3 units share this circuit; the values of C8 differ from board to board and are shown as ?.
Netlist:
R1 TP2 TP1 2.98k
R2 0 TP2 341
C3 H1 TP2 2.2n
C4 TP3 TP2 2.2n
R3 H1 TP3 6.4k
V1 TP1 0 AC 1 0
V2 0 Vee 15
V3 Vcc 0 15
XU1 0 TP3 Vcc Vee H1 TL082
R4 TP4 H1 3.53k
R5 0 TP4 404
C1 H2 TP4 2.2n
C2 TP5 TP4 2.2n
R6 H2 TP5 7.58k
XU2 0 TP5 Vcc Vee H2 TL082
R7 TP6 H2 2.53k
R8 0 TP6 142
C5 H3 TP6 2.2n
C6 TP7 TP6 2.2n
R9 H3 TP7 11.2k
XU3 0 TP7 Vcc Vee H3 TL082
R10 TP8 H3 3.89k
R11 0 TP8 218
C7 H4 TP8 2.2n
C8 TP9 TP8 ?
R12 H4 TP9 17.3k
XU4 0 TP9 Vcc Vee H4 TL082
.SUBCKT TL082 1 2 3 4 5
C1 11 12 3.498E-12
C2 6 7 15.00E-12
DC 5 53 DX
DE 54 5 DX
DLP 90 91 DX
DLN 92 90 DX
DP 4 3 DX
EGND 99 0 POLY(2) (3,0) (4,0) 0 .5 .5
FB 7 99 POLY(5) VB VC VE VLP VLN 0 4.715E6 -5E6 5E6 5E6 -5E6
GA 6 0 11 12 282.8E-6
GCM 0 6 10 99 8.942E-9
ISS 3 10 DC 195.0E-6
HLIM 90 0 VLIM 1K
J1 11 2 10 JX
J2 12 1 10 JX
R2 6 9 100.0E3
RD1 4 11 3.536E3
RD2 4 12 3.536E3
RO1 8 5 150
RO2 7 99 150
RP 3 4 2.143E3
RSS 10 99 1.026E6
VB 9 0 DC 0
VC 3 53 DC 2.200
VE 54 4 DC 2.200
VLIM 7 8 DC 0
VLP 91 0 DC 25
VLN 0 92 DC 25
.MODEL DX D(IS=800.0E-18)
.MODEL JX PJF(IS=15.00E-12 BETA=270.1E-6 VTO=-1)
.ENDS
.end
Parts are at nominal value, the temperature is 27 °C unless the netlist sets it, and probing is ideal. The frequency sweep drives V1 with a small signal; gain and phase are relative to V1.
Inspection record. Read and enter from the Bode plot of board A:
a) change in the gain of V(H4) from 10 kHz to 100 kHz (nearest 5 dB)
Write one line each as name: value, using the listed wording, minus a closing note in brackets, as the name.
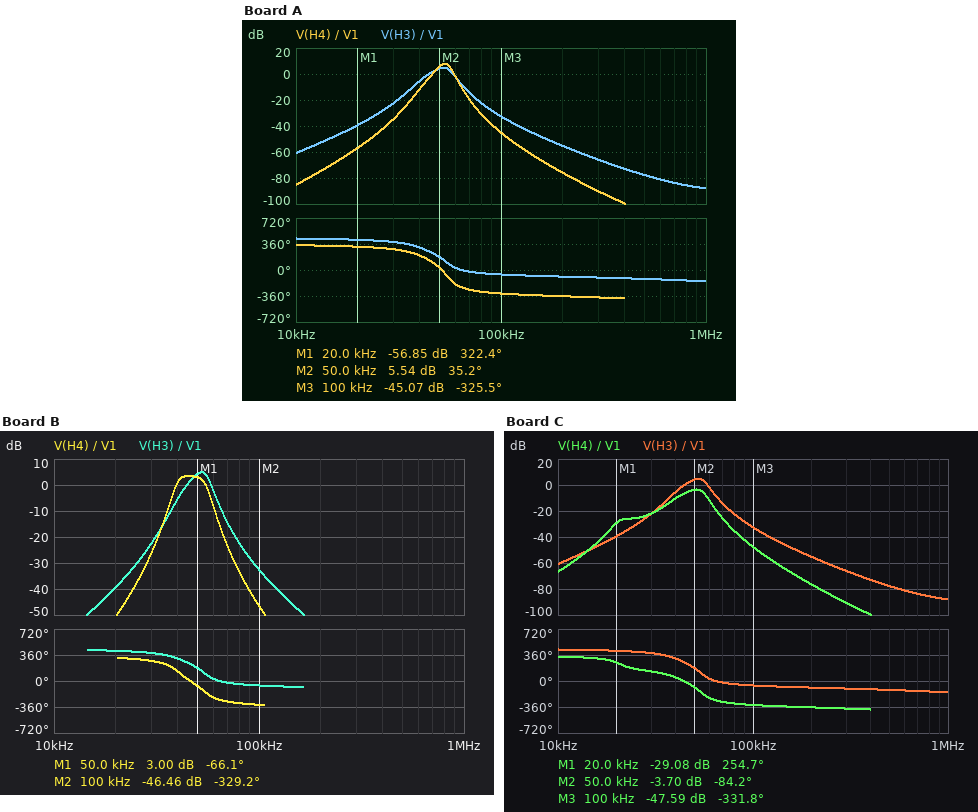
change in the gain of V(H4) from 10 kHz to 100 kHz: 40 dB
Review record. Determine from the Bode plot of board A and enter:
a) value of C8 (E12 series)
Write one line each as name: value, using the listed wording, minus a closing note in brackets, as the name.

value of C8: 1 nF
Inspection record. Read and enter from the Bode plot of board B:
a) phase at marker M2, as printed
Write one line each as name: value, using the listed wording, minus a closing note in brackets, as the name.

phase at marker M2, as printed: -329.2 deg
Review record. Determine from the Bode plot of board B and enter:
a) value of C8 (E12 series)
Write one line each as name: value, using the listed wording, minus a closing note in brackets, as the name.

value of C8: 1.8 nF
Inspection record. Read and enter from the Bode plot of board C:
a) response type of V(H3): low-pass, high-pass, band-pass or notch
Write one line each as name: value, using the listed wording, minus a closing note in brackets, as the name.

response type of V(H3): low-pass, high-pass, band-pass or notch: band-pass
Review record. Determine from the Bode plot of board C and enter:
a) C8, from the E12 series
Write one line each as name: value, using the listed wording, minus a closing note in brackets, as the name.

C8, from the E12 series: 6.8 nF
